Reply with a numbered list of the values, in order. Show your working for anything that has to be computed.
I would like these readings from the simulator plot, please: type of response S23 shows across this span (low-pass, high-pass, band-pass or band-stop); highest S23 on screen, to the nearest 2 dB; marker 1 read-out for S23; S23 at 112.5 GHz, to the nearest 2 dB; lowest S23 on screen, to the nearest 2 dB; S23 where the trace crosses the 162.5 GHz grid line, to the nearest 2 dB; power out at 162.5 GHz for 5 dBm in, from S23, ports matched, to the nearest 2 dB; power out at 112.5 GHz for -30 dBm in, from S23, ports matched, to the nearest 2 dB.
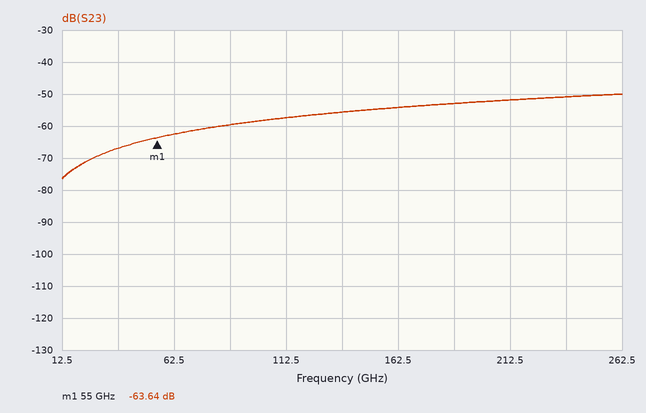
1. high-pass
2. -50 dB
3. -63.64 dB
4. -58 dB
5. -76 dB
6. -54 dB
7. 5 dBm + (-54 dB) = -50 dBm
8. -30 dBm + (-58 dB) = -88 dBm
